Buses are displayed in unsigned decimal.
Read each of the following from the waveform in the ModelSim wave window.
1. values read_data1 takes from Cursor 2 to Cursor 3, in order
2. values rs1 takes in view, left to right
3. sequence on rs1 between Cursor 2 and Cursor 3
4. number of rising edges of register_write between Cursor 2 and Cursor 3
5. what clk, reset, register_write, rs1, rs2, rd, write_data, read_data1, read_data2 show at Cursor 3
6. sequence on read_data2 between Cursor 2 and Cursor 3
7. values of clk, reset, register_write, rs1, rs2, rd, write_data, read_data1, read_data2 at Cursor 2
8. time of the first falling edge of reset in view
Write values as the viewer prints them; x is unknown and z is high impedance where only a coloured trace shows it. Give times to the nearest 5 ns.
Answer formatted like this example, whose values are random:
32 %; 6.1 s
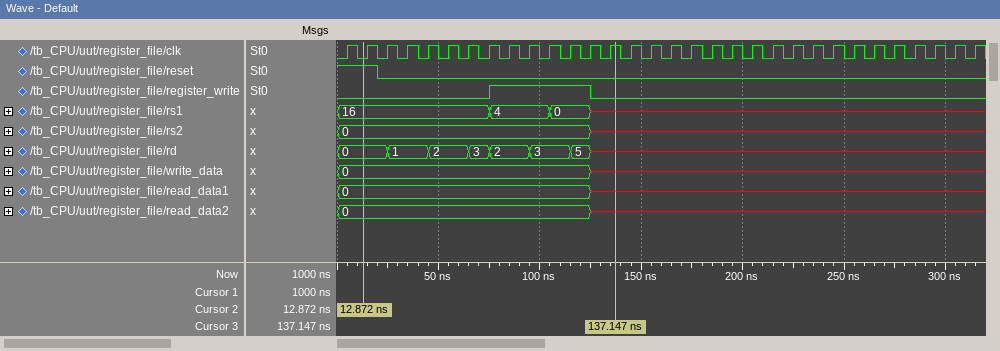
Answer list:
0, x; 16, 4, 0, x; 16, 4, 0, x; 1; clk=1, reset=0, register_write=0, rs1=x, rs2=x, rd=x, write_data=x, read_data1=x, read_data2=x; 0, x; clk=0, reset=1, register_write=0, rs1=16, rs2=0, rd=0, write_data=0, read_data1=0, read_data2=0; 20 ns
